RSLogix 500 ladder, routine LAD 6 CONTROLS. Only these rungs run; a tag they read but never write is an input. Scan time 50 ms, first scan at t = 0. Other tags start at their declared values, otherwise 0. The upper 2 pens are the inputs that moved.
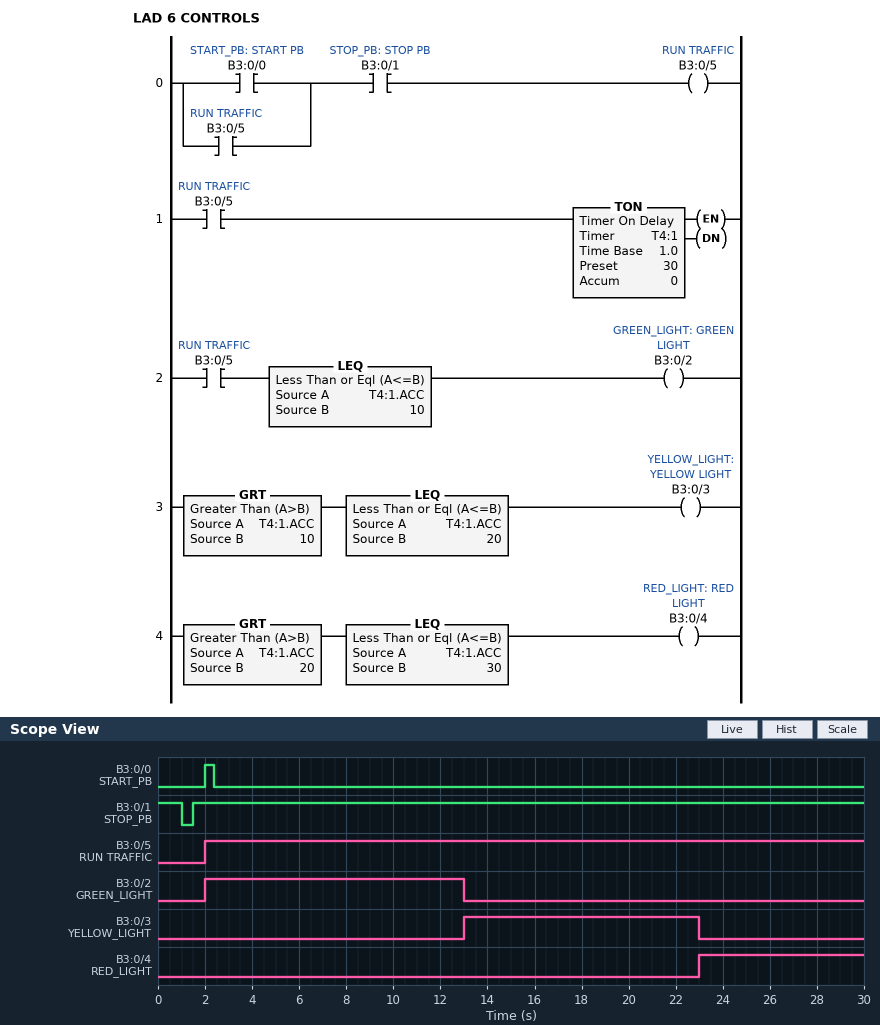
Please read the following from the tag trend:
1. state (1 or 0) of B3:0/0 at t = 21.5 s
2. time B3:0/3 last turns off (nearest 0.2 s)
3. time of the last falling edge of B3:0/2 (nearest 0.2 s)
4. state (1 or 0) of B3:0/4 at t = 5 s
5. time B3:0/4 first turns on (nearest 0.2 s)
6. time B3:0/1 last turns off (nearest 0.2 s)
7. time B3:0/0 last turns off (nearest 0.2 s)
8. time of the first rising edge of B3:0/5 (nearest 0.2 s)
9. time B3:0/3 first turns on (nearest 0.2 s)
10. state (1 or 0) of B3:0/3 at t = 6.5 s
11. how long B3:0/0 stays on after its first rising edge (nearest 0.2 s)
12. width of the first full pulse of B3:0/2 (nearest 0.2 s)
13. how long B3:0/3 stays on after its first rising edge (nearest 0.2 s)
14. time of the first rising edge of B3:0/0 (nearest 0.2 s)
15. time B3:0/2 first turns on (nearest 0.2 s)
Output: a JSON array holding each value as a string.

["0", "23.0 s", "13.0 s", "0", "23.0 s", "1.0 s", "2.4 s", "2.0 s", "13.0 s", "0", "0.4 s", "11.0 s", "10.0 s", "2.0 s", "2.0 s"]
